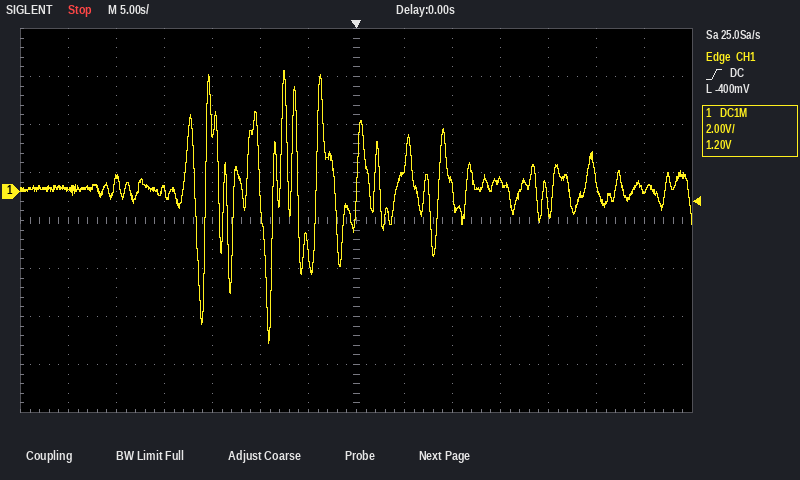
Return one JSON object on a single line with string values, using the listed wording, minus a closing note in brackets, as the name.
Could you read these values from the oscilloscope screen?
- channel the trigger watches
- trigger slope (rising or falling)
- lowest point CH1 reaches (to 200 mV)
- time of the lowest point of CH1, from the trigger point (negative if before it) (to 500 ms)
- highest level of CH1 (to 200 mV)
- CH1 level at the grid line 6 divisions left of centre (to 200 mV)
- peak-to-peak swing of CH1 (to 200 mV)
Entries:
{"channel the trigger watches": "CH1", "trigger slope": "rising", "lowest point CH1 reaches": "-6.4 V", "time of the lowest point of CH1, from the trigger point (negative if before it)": "-9.0 s", "highest level of CH1": "5.0 V", "CH1 level at the grid line 6 divisions left of centre": "0.0 V", "peak-to-peak swing of CH1": "11.4 V"}
